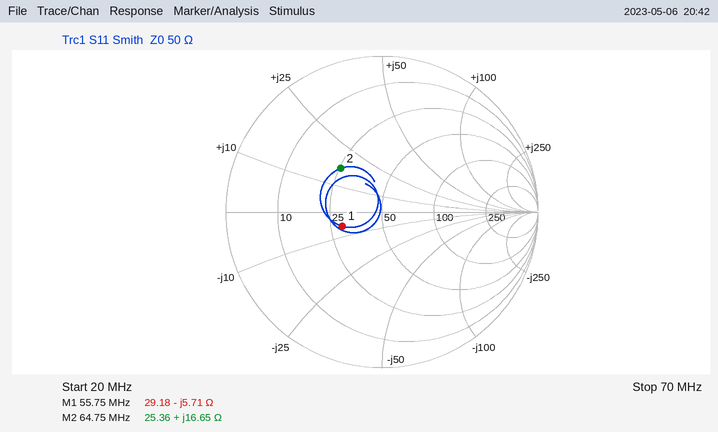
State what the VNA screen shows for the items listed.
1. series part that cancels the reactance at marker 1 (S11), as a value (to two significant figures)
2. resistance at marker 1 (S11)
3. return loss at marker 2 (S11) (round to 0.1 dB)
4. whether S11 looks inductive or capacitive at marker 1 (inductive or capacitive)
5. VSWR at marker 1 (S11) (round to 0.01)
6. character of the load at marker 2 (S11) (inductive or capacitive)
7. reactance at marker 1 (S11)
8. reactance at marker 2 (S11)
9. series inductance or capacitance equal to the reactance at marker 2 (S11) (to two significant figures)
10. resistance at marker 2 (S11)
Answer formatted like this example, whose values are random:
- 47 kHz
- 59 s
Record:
- 16 nH
- 29.18 Ω
- 8.3 dB
- capacitive
- 1.75
- inductive
- -5.71 Ω
- +16.65 Ω
- 41 nH
- 25.36 Ω
